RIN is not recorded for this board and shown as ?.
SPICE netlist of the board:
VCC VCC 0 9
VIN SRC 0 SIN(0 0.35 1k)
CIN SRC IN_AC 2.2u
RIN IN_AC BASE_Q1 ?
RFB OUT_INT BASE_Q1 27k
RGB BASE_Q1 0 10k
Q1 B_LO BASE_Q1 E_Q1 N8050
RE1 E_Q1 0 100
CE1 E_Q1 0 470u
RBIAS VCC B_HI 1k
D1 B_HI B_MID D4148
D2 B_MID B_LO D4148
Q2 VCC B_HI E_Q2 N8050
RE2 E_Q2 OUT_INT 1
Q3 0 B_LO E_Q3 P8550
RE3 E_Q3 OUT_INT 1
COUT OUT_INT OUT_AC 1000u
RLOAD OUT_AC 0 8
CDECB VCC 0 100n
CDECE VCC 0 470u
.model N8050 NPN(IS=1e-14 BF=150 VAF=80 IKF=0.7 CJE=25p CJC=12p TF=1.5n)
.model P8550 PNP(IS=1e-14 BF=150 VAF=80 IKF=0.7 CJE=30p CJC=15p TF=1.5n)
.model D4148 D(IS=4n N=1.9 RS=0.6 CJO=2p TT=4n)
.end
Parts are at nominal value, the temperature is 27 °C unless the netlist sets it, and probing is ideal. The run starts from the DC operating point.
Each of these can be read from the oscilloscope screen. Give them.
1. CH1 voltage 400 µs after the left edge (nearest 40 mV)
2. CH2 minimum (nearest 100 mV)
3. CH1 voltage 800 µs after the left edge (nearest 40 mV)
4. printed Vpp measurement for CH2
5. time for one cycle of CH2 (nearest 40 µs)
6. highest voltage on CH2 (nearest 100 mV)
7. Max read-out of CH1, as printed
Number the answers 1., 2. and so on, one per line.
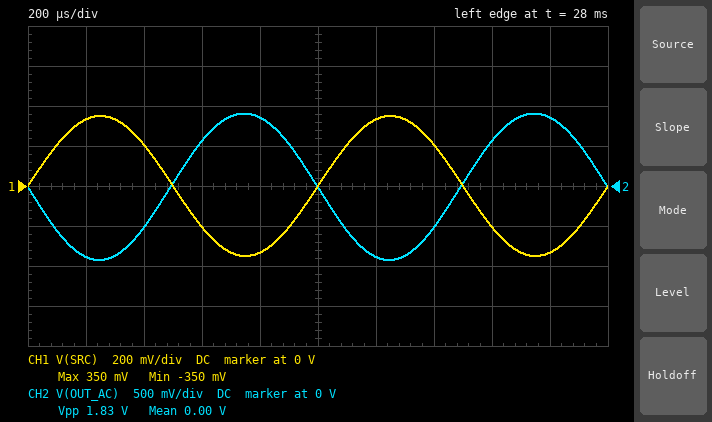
1. 200 mV
2. -900 mV
3. -320 mV
4. 1.83 V
5. 1.00 ms
6. 900 mV
7. 350 mV
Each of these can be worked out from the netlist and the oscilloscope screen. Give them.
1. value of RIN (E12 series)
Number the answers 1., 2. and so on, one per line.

1. 6.8 kΩ
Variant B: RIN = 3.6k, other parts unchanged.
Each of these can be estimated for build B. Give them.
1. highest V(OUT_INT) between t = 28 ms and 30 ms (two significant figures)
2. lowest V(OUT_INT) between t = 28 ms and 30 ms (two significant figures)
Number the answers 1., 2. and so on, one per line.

1. 6.1 V
2. 2.9 V
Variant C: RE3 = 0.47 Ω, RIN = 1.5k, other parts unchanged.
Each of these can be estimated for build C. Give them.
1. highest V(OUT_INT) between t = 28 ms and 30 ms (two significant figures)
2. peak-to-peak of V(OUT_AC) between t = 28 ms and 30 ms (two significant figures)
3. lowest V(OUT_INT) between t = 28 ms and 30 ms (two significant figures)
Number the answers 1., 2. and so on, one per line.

1. 6.2 V
2. 4.6 V
3. 1.6 V
